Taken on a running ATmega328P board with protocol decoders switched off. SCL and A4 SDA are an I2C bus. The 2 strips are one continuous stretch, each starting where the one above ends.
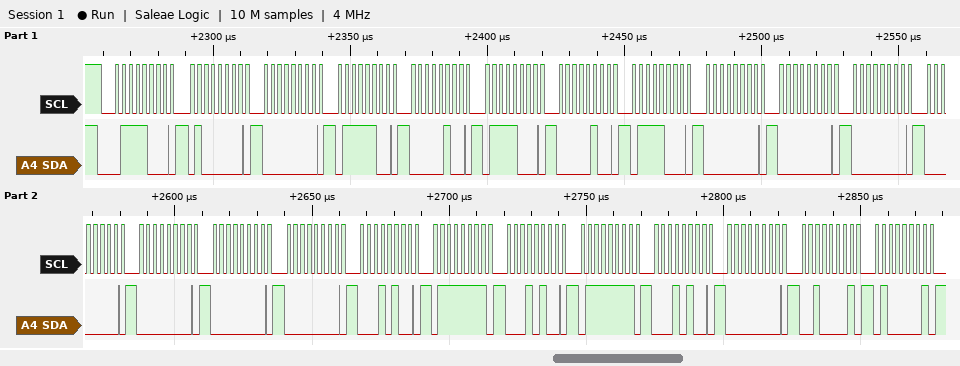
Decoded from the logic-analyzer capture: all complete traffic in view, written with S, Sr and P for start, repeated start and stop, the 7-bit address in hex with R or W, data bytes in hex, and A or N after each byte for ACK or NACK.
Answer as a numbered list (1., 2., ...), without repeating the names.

1. S 3CW A 40 A 00 A 7C A 04 A 78 A 04 A 78 A 00 A 00 A 00 A 00 A 00 A 00 A 00 A 14 A 7F A 14 A 7F A 14 A 00 A 21 A 41 A
